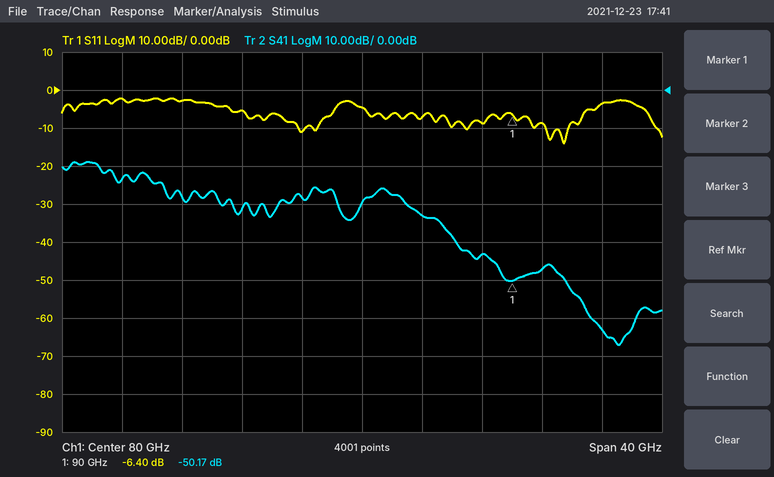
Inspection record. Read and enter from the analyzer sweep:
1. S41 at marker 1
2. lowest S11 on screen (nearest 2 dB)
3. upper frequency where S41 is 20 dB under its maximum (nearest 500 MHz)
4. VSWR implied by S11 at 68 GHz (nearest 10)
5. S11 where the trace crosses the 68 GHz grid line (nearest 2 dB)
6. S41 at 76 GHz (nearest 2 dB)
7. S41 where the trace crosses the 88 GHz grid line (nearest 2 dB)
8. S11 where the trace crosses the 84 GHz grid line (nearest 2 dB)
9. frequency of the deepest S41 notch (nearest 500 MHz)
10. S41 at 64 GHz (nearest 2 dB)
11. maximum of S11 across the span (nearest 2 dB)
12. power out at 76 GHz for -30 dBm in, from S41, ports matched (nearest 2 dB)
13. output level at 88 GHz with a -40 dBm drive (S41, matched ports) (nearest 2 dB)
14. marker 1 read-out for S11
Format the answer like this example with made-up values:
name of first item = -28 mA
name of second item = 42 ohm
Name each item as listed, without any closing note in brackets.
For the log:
S41 at marker 1 = -50.17 dB
lowest S11 on screen = -14 dB
upper frequency where S41 is 20 dB under its maximum = 86.0 GHz
VSWR implied by S11 at 68 GHz = 10
S11 where the trace crosses the 68 GHz grid line = -2 dB
S41 at 76 GHz = -28 dB
S41 where the trace crosses the 88 GHz grid line = -44 dB
S11 where the trace crosses the 84 GHz grid line = -8 dB
frequency of the deepest S41 notch = 97.0 GHz
S41 at 64 GHz = -24 dB
maximum of S11 across the span = -2 dB
power out at 76 GHz for -30 dBm in, from S41, ports matched = -58 dBm
output level at 88 GHz with a -40 dBm drive (S41, matched ports) = -84 dBm
marker 1 read-out for S11 = -6.40 dB
